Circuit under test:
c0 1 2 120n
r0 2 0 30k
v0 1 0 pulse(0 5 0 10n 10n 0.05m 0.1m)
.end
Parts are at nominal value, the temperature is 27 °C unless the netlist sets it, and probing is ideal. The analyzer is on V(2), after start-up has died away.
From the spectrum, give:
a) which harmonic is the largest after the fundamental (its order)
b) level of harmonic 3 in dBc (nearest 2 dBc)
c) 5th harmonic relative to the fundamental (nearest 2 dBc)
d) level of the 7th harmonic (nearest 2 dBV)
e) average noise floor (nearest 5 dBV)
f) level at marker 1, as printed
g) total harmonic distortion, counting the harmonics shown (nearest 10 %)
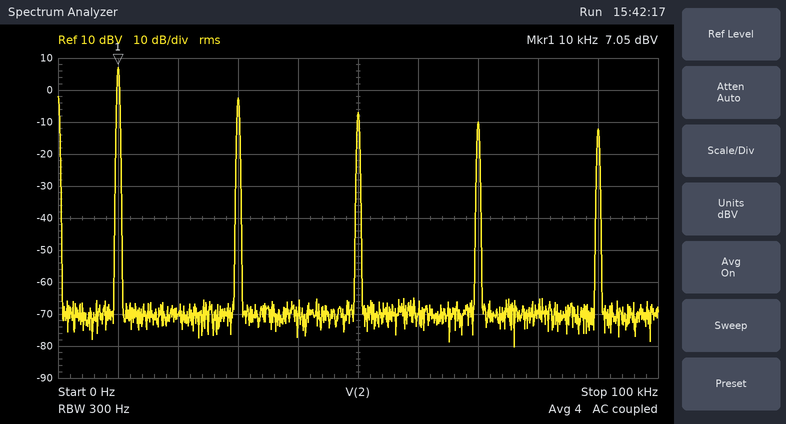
3
-10 dBc
-14 dBc
-10 dBV
-70 dBV
7.05 dBV
40 %
